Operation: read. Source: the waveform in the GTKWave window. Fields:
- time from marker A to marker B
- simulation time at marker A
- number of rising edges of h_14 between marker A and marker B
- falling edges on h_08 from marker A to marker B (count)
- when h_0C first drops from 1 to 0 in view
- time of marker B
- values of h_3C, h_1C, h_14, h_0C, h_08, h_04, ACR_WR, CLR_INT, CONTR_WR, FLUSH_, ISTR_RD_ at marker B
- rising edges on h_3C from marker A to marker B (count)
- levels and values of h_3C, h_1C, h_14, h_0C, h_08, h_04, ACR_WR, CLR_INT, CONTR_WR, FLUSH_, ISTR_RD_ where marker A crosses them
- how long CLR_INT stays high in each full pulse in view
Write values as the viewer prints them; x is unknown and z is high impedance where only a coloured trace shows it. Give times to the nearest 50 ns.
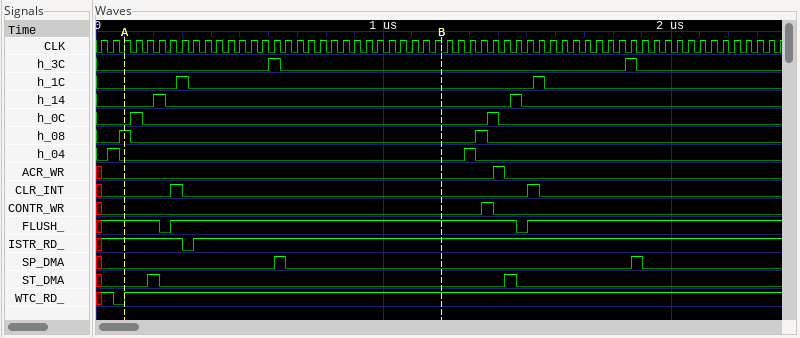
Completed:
1100 ns
100 ns
1
1
150 ns
1200 ns
h_3C=0, h_1C=0, h_14=0, h_0C=0, h_08=0, h_04=0, ACR_WR=0, CLR_INT=0, CONTR_WR=0, FLUSH_=1, ISTR_RD_=1
1
h_3C=0, h_1C=0, h_14=0, h_0C=0, h_08=1, h_04=0, ACR_WR=0, CLR_INT=0, CONTR_WR=0, FLUSH_=1, ISTR_RD_=1
50 ns, 50 ns
